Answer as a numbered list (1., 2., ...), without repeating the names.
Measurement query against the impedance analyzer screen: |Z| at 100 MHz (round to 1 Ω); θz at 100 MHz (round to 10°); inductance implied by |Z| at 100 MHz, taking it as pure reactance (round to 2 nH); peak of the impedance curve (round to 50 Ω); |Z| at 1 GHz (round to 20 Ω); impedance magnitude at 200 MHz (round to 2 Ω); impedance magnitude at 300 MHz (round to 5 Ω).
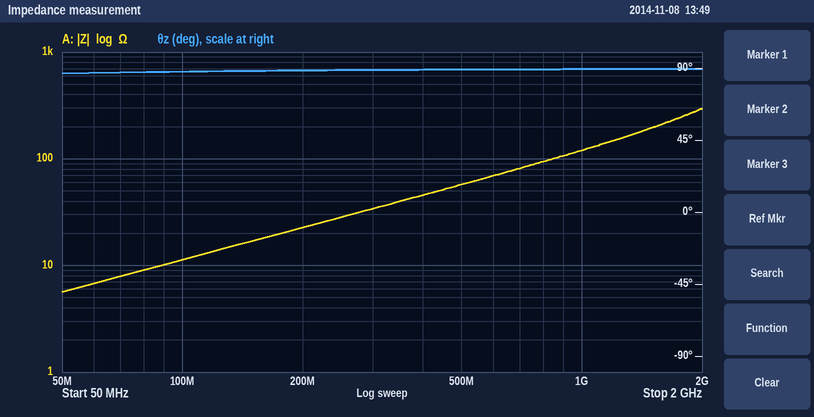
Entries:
1. 11 Ω
2. 90°
3. 18 nH
4. 300 Ω
5. 120 Ω
6. 22 Ω
7. 35 Ω
